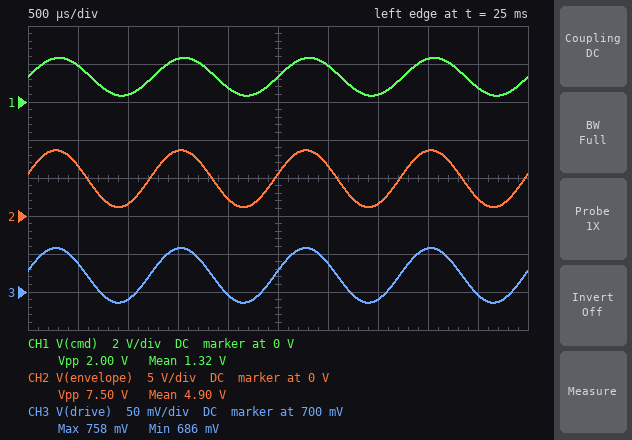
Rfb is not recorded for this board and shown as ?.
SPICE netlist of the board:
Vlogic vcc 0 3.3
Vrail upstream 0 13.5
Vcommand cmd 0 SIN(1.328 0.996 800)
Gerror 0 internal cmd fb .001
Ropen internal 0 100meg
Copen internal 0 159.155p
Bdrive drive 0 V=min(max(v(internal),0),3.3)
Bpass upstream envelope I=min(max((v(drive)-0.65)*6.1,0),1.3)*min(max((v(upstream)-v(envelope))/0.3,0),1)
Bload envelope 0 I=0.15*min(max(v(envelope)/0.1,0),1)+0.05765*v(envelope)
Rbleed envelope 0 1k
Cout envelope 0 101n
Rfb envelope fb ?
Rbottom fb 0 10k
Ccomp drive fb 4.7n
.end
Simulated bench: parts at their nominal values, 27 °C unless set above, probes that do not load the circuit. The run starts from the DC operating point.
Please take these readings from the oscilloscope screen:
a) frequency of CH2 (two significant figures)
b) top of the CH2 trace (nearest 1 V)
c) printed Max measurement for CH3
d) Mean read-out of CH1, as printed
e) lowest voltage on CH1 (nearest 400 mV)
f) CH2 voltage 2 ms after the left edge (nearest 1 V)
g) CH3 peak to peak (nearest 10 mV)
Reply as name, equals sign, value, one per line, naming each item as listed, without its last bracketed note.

frequency of CH2 = 800 Hz
top of the CH2 trace = 9 V
printed Max measurement for CH3 = 758 mV
Mean read-out of CH1, as printed = 1.32 V
lowest voltage on CH1 = 400 mV
CH2 voltage 2 ms after the left edge = 2 V
CH3 peak to peak = 70 mV
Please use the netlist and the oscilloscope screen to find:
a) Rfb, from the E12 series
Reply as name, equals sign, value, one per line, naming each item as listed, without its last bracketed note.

Rfb, from the E12 series = 27 kΩ
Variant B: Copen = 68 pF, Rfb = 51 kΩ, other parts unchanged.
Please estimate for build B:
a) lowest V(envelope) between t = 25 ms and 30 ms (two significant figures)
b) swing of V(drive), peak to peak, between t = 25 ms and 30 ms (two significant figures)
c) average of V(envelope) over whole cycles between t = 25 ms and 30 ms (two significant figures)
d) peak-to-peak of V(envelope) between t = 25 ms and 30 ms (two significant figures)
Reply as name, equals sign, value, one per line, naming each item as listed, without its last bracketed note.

lowest V(envelope) between t = 25 ms and 30 ms = 1.9 V
swing of V(drive), peak to peak, between t = 25 ms and 30 ms = 760 mV
average of V(envelope) over whole cycles between t = 25 ms and 30 ms = 8.1 V
peak-to-peak of V(envelope) between t = 25 ms and 30 ms = 11 V
